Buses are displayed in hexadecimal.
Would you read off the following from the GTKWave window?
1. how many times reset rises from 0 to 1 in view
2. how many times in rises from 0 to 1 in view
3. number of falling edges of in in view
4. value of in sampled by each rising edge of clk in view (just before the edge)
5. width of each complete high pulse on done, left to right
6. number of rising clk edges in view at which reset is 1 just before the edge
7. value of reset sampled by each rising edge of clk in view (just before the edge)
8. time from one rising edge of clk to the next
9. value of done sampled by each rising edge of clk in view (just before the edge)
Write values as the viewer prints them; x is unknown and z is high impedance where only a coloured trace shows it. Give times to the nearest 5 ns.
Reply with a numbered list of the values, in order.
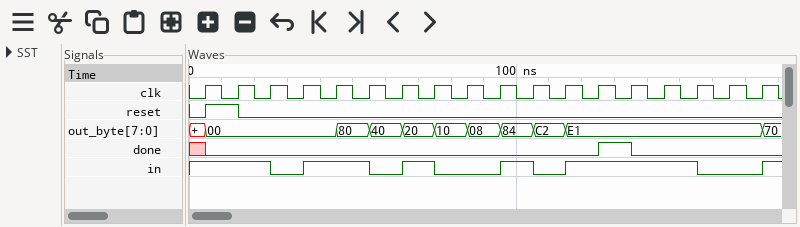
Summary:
1. 1
2. 5
3. 5
4. 1 1 1 0 1 1 0 1 0 0 1 0 1 1 1 1 0 0
5. 10 ns
6. 1
7. 0 1 0 0 0 0 0 0 0 0 0 0 0 0 0 0 0 0
8. 10 ns
9. x 0 0 0 0 0 0 0 0 0 0 0 0 1 0 0 0 0
